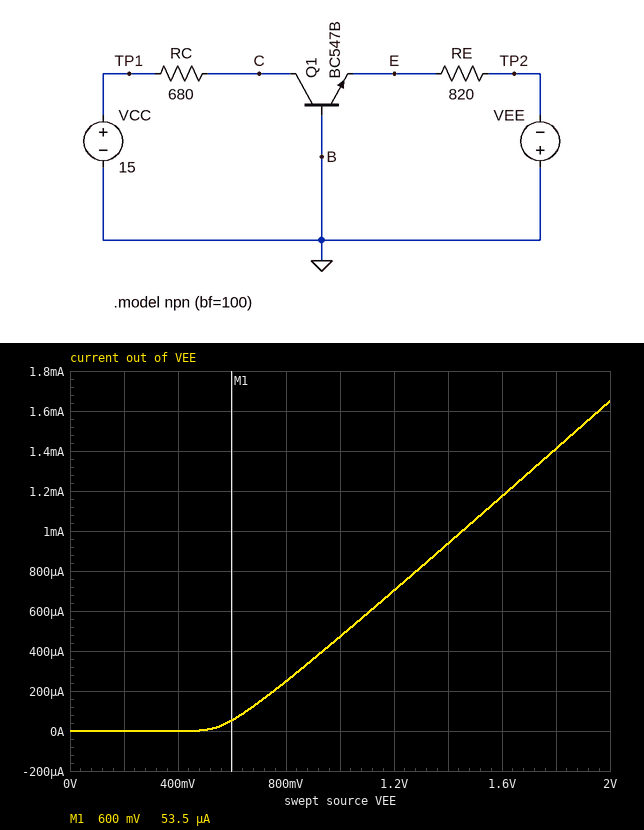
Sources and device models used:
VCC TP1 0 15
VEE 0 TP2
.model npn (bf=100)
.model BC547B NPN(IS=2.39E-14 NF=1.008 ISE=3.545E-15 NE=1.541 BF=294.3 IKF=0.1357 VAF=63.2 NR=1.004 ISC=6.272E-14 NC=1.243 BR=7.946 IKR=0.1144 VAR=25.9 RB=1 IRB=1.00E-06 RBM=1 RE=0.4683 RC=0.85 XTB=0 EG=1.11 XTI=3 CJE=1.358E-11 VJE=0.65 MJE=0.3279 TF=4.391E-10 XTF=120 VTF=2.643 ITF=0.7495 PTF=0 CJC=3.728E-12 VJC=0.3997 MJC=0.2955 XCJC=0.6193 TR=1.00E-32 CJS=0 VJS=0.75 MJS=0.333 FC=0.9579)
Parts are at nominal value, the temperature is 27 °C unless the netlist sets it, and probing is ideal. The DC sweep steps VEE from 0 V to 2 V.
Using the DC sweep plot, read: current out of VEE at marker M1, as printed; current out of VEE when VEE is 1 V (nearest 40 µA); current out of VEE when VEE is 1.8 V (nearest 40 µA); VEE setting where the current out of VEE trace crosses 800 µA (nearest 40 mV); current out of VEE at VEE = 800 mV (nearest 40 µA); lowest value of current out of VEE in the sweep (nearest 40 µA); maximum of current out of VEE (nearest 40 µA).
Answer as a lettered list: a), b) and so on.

a) 53.5 µA
b) 480 µA
c) 1.40 mA
d) 1.28 V
e) 240 µA
f) 0 A
g) 1.64 mA
